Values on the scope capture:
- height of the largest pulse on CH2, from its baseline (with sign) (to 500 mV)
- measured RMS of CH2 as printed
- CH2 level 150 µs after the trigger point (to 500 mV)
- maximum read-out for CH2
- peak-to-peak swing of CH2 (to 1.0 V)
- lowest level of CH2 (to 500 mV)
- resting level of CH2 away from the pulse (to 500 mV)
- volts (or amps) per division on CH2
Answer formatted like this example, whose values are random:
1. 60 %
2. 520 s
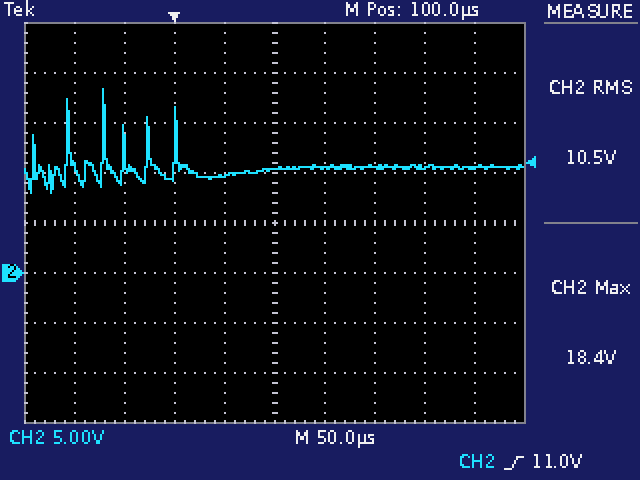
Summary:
1. +8.0 V
2. 10.5 V
3. 10.5 V
4. 18.4 V
5. 10.0 V
6. 8.0 V
7. 10.5 V
8. 5 V
